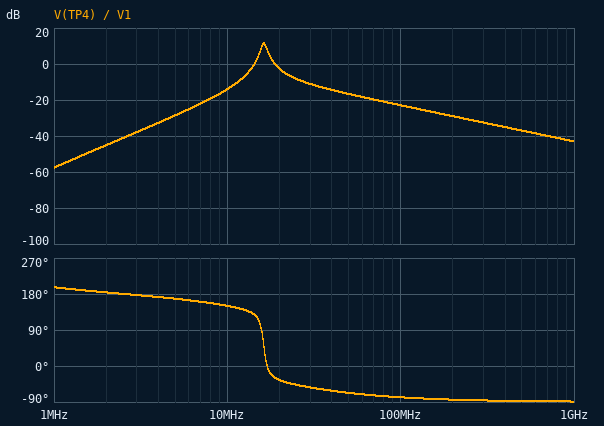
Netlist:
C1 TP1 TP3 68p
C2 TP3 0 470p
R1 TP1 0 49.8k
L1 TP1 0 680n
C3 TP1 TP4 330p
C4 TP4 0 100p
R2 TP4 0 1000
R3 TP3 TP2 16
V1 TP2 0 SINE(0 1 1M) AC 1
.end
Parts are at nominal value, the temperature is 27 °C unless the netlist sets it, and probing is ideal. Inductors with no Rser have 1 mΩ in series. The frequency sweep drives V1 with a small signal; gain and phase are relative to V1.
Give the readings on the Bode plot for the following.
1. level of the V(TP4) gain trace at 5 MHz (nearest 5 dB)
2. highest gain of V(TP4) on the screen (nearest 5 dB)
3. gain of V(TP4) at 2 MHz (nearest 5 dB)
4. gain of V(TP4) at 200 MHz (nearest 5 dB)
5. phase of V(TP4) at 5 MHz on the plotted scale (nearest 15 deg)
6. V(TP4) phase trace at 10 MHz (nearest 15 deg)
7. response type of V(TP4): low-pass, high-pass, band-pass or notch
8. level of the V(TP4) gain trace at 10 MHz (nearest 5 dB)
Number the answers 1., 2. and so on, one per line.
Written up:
1. -30 dB
2. 10 dB
3. -45 dB
4. -30 dB
5. 165 deg
6. 150 deg
7. band-pass
8. -15 dB
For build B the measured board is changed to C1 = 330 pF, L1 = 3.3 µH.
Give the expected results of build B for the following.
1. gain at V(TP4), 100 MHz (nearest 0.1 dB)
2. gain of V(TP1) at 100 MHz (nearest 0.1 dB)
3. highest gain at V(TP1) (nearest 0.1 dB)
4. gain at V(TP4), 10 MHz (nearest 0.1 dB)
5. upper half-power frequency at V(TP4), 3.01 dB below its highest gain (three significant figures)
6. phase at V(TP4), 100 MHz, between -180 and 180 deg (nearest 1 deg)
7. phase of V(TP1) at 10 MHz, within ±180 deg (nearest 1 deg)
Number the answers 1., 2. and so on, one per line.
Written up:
1. -18.8 dB
2. -16.5 dB
3. 13.6 dB
4. -3.3 dB
5. 4.84 MHz
6. -79 deg
7. -23 deg
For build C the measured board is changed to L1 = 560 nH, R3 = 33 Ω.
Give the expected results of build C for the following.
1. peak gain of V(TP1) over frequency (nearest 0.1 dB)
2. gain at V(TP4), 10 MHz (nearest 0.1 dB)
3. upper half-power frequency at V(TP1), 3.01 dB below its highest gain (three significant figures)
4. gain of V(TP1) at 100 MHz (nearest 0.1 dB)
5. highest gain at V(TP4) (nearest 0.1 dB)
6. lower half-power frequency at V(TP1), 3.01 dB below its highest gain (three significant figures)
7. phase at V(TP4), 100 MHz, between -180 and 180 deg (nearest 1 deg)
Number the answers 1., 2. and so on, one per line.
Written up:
1. 10.7 dB
2. -19.1 dB
3. 18.7 MHz
4. -26.7 dB
5. 8.4 dB
6. 17.5 MHz
7. -84 deg
